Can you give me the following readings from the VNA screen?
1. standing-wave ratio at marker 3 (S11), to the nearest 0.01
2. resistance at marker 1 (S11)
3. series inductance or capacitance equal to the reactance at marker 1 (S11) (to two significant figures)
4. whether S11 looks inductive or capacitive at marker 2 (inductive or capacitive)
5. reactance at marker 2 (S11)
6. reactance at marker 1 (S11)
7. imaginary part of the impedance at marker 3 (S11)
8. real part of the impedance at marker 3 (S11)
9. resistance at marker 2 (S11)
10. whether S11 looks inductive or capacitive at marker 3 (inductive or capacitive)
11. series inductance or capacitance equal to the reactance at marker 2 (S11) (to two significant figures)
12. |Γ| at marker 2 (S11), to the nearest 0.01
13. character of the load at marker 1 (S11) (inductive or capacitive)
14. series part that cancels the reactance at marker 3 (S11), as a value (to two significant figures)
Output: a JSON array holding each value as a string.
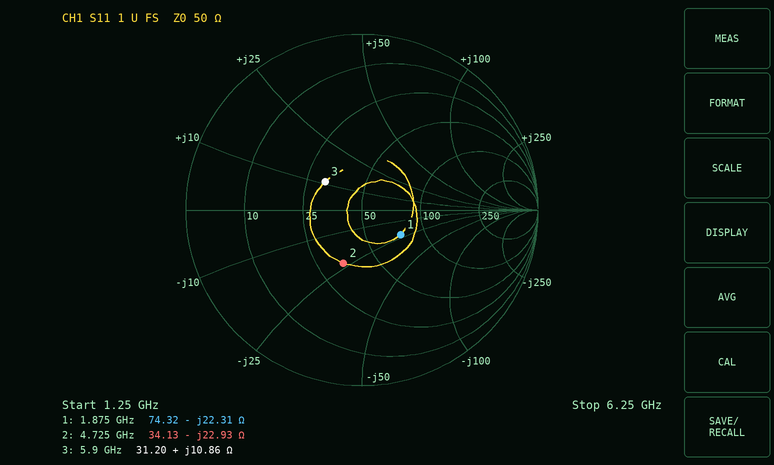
["1.72", "74.32 Ω", "3.8 pF", "capacitive", "-22.93 Ω", "-22.31 Ω", "+10.86 Ω", "31.20 Ω", "34.13 Ω", "inductive", "1.5 pF", "0.32", "capacitive", "2.5 pF"]
